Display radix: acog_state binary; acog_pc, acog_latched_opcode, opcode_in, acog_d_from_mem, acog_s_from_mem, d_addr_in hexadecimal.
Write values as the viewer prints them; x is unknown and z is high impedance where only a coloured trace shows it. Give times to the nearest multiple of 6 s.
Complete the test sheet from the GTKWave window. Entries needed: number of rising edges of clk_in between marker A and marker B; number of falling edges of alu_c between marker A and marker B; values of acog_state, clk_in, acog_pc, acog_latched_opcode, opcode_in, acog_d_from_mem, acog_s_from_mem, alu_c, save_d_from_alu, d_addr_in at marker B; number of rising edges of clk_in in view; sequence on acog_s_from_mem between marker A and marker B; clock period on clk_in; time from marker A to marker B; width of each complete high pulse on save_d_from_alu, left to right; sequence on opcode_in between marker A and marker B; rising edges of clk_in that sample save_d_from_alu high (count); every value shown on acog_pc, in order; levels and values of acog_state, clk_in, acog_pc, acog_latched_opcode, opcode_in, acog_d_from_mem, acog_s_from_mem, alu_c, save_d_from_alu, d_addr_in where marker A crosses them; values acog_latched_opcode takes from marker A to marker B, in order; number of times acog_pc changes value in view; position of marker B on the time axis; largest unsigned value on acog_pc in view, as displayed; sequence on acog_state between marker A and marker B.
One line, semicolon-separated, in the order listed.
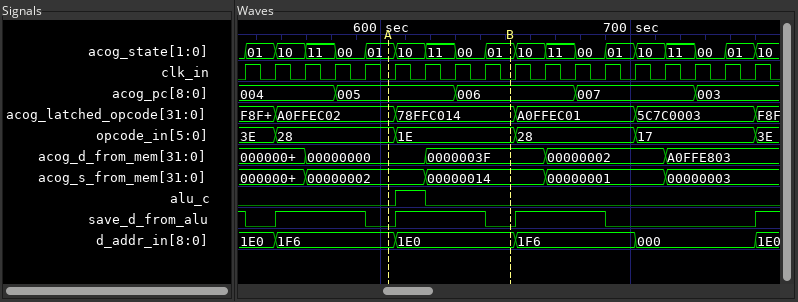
4; 1; acog_state=01, clk_in=0, acog_pc=006, acog_latched_opcode=78FFC014, opcode_in=1E, acog_d_from_mem=0000003F, acog_s_from_mem=00000014, alu_c=0, save_d_from_alu=0, d_addr_in=1E0; 18; 00000002, 00000014; 12 s; 48 s; 36 s, 36 s, 36 s; 28, 1E; 10; 004, 005, 006, 007, 003; acog_state=01, clk_in=0, acog_pc=005, acog_latched_opcode=A0FFEC02, opcode_in=28, acog_d_from_mem=00000000, acog_s_from_mem=00000002, alu_c=0, save_d_from_alu=0, d_addr_in=1F6; A0FFEC02, 78FFC014; 4; 654 s; 007; 01, 10, 11, 00, 01
